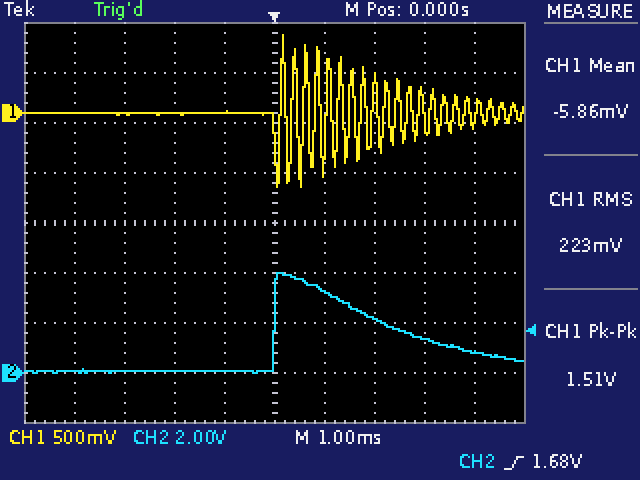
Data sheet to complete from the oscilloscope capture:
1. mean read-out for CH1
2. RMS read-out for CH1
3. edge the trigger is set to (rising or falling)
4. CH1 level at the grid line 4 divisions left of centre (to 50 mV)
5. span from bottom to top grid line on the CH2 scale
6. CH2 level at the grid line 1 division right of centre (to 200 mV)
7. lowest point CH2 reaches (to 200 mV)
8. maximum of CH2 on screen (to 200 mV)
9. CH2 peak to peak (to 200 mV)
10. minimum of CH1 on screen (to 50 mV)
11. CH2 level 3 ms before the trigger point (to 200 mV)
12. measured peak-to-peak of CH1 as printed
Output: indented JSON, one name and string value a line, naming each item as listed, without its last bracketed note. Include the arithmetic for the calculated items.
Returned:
{
  "mean read-out for CH1": "-5.86 mV",
  "RMS read-out for CH1": "223 mV",
  "edge the trigger is set to": "rising",
  "CH1 level at the grid line 4 divisions left of centre": "0 mV",
  "span from bottom to top grid line on the CH2 scale": "16 V",
  "CH2 level at the grid line 1 division right of centre": "3.2 V",
  "lowest point CH2 reaches": "0.0 V",
  "maximum of CH2 on screen": "4.0 V",
  "CH2 peak to peak": "4.0 V − (0.0 V) = 4.0 V",
  "minimum of CH1 on screen": "-750 mV",
  "CH2 level 3 ms before the trigger point": "0.0 V",
  "measured peak-to-peak of CH1 as printed": "1.51 V"
}
